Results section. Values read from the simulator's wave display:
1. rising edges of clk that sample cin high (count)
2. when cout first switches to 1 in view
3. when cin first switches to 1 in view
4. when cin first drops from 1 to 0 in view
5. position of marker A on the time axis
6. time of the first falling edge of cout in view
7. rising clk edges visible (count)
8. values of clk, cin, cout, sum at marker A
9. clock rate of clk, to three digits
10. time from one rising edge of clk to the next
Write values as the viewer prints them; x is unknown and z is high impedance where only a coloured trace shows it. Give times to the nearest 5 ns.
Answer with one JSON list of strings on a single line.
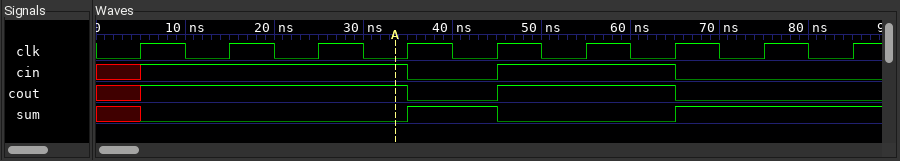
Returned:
["5", "5 ns", "5 ns", "35 ns", "35 ns", "35 ns", "9", "clk=0, cin=1, cout=1, sum=0", "100 MHz", "10 ns"]
